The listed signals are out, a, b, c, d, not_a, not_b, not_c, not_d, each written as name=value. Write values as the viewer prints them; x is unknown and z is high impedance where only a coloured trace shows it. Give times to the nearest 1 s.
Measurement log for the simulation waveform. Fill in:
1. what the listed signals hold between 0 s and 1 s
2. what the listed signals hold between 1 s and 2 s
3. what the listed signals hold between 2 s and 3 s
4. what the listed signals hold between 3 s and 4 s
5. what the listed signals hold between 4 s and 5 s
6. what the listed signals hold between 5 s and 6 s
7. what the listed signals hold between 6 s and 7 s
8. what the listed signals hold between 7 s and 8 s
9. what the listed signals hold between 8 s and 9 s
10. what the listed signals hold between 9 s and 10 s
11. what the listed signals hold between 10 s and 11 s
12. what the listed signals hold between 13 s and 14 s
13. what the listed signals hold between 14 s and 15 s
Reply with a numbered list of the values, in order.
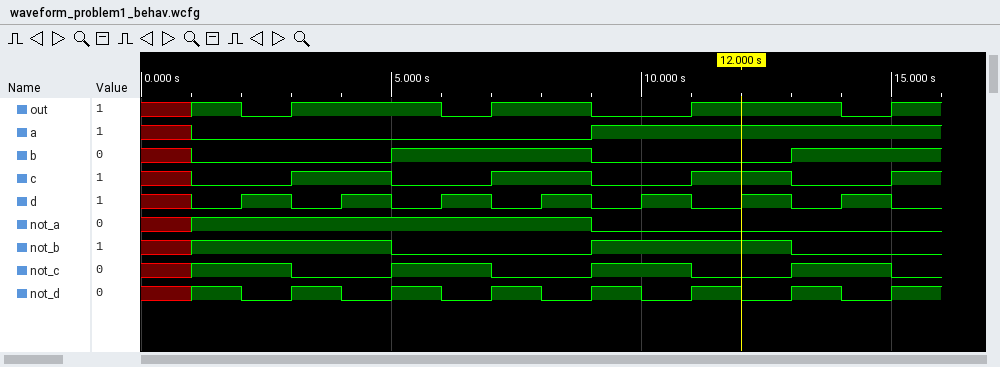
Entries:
1. out=x, a=x, b=x, c=x, d=x, not_a=x, not_b=x, not_c=x, not_d=x
2. out=1, a=0, b=0, c=0, d=0, not_a=1, not_b=1, not_c=1, not_d=1
3. out=0, a=0, b=0, c=0, d=1, not_a=1, not_b=1, not_c=1, not_d=0
4. out=1, a=0, b=0, c=1, d=0, not_a=1, not_b=1, not_c=0, not_d=1
5. out=1, a=0, b=0, c=1, d=1, not_a=1, not_b=1, not_c=0, not_d=0
6. out=1, a=0, b=1, c=0, d=0, not_a=1, not_b=0, not_c=1, not_d=1
7. out=0, a=0, b=1, c=0, d=1, not_a=1, not_b=0, not_c=1, not_d=0
8. out=1, a=0, b=1, c=1, d=0, not_a=1, not_b=0, not_c=0, not_d=1
9. out=1, a=0, b=1, c=1, d=1, not_a=1, not_b=0, not_c=0, not_d=0
10. out=0, a=1, b=0, c=0, d=0, not_a=0, not_b=1, not_c=1, not_d=1
11. out=0, a=1, b=0, c=0, d=1, not_a=0, not_b=1, not_c=1, not_d=0
12. out=1, a=1, b=1, c=0, d=0, not_a=0, not_b=0, not_c=1, not_d=1
13. out=0, a=1, b=1, c=0, d=1, not_a=0, not_b=0, not_c=1, not_d=0
